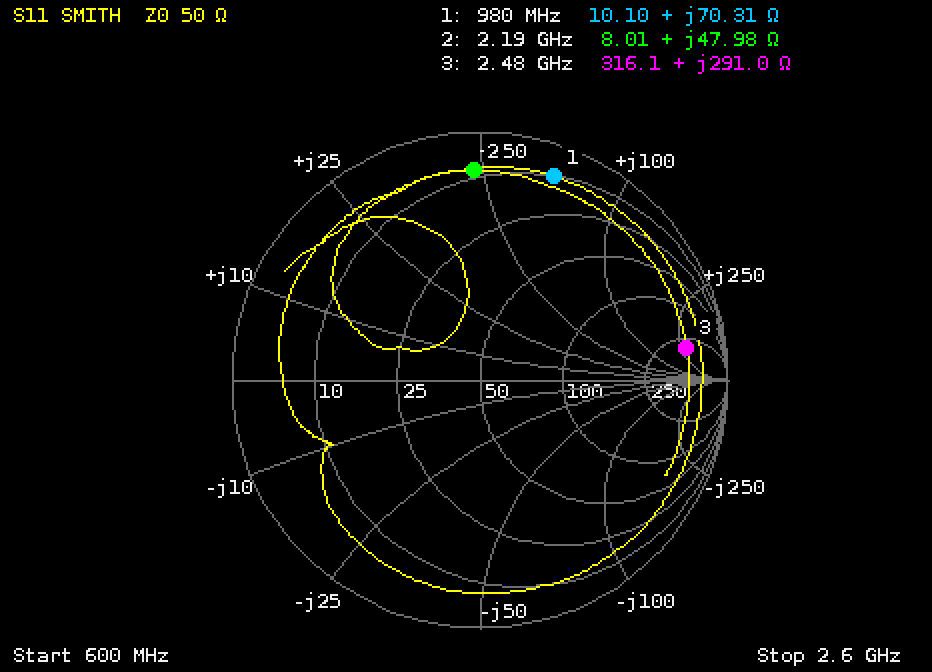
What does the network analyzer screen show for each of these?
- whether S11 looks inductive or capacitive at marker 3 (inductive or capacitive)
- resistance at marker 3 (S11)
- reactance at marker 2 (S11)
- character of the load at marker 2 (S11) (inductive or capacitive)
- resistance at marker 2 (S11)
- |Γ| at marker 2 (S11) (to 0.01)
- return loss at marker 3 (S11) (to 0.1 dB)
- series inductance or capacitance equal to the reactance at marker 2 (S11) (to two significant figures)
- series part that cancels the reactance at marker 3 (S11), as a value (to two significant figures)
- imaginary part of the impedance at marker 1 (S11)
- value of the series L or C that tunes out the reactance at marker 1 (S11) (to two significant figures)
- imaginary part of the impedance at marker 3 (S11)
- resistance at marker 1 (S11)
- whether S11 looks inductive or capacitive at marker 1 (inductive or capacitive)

inductive
316.1 Ω
+47.98 Ω
inductive
8.01 Ω
0.85
1.5 dB
3.5 nH
220 fF
+70.31 Ω
2.3 pF
+291.0 Ω
10.10 Ω
inductive
